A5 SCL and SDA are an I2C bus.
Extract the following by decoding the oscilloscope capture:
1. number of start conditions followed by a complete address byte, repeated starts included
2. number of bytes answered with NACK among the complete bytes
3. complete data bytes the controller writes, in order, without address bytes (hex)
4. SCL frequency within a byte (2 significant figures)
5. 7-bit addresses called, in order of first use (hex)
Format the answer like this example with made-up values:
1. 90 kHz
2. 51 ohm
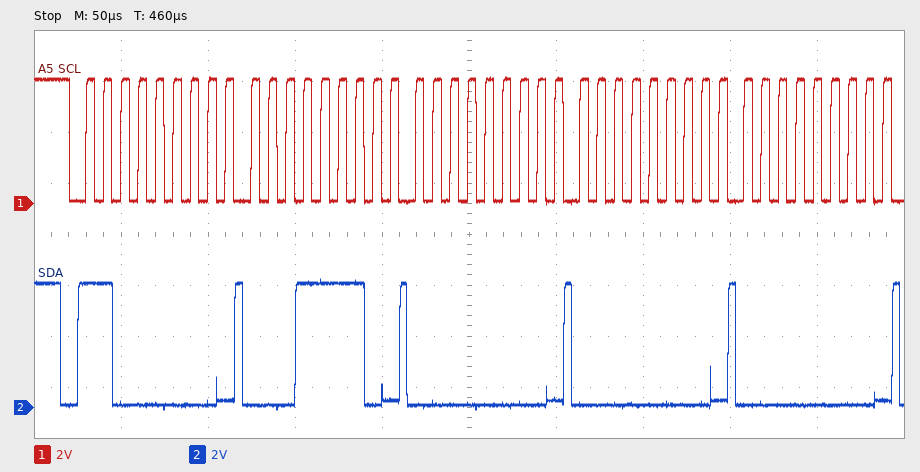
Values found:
1. 1
2. 0
3. 1E 00 00 00
4. 100 kHz
5. 0x60
